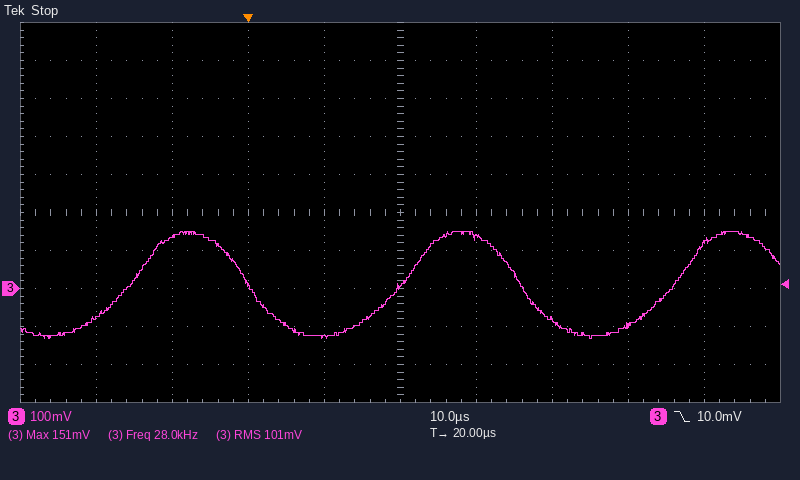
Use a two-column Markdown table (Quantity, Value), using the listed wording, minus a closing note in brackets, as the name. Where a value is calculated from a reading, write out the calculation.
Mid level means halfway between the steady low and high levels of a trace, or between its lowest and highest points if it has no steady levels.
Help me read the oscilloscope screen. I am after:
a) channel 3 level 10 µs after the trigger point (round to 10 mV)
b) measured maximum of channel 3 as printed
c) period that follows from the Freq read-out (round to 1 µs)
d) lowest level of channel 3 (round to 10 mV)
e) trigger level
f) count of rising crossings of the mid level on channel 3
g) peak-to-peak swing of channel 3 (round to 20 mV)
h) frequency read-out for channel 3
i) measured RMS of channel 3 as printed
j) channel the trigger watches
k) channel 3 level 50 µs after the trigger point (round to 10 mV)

| Quantity | Value |
|---|---|
| channel 3 level 10 µs after the trigger point | -130 mV |
| measured maximum of channel 3 as printed | 151 mV |
| period that follows from the Freq read-out | 1 / 28.0 kHz ≈ 36 µs |
| lowest level of channel 3 | -130 mV |
| trigger level | 10.0 mV |
| count of rising crossings of the mid level on channel 3 | 3 |
| peak-to-peak swing of channel 3 | 280 mV |
| frequency read-out for channel 3 | 28.0 kHz |
| measured RMS of channel 3 as printed | 101 mV |
| channel the trigger watches | channel 3 |
| channel 3 level 50 µs after the trigger point | -100 mV |
